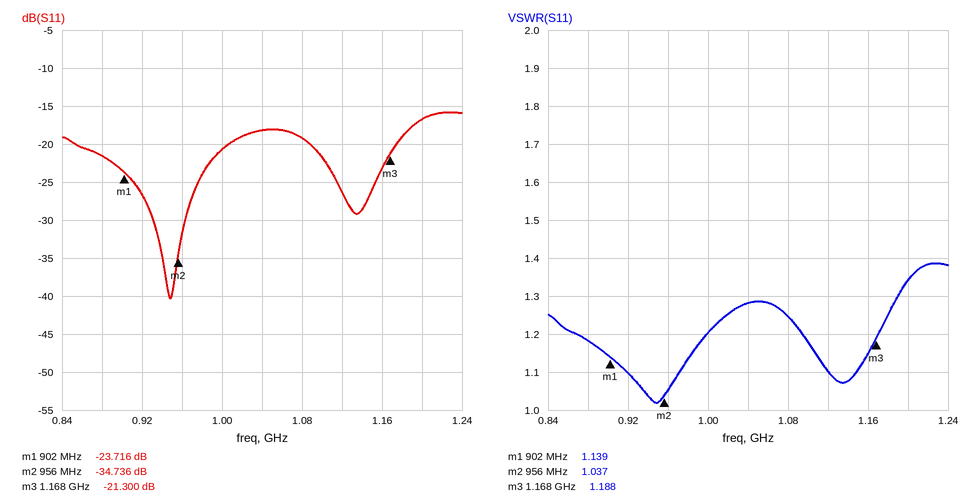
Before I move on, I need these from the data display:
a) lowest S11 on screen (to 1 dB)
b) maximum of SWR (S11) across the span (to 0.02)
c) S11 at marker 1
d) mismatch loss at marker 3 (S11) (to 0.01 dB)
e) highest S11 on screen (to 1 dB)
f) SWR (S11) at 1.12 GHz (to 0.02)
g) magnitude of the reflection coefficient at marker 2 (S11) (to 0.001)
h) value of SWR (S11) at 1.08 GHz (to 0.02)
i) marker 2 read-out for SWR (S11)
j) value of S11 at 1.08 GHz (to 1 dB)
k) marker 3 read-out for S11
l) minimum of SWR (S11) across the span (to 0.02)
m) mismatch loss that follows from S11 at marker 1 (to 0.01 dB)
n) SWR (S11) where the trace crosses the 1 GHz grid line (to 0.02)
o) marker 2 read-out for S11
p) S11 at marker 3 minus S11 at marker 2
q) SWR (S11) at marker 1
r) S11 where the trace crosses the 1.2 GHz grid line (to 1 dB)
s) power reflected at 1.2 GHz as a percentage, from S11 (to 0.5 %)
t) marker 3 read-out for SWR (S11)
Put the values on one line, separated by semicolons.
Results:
-40 dB; 1.38; -23.716 dB; 0.03 dB; -16 dB; 1.10; 0.018; 1.24; 1.037; -19 dB; -21.300 dB; 1.02; 0.02 dB; 1.20; -34.736 dB; 13.436 dB; 1.139; -17 dB; 2.0 %; 1.188
